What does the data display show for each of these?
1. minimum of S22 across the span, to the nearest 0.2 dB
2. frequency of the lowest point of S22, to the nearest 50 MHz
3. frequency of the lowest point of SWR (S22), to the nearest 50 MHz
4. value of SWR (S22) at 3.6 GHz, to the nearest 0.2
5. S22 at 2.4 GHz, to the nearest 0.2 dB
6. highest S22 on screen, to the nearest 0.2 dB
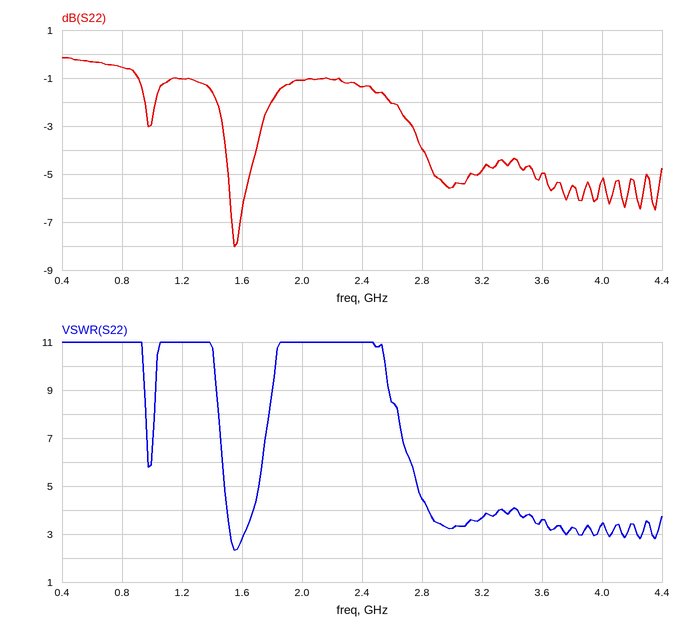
-8.0 dB
1.55 GHz
1.55 GHz
3.6
-1.4 dB
-0.2 dB
